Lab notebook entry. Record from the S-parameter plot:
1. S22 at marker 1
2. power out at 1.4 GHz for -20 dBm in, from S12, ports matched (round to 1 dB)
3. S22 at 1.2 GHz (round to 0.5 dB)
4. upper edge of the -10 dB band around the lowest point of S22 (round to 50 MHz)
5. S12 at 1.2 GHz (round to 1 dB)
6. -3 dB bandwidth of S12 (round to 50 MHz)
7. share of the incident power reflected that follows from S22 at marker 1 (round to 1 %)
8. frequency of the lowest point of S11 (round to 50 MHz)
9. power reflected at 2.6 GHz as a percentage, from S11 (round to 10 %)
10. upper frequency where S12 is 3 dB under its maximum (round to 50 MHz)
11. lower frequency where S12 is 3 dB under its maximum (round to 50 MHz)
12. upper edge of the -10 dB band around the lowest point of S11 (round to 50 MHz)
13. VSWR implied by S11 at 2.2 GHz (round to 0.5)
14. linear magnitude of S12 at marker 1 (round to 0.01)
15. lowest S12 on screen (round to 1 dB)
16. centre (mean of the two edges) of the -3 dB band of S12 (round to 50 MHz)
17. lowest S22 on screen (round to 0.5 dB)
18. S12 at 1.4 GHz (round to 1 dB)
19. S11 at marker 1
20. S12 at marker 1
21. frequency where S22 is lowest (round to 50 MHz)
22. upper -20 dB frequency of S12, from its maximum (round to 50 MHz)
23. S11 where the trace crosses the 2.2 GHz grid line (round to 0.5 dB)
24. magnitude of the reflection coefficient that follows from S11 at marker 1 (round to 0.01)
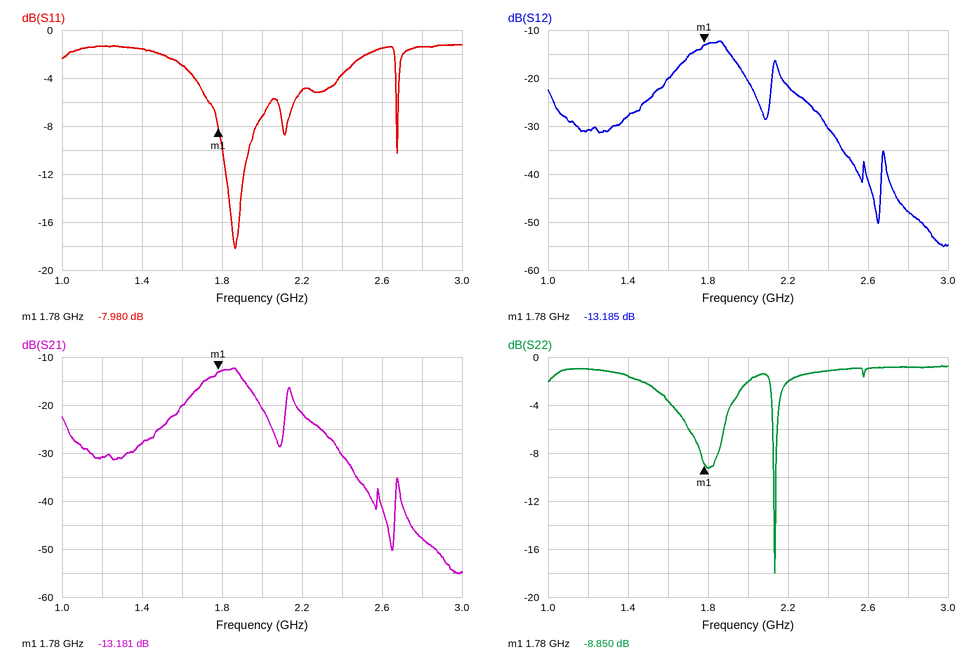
-8.850 dB
-48 dBm
-1.0 dB
2.15 GHz
-31 dB
200 MHz
13 %
1.85 GHz
70 %
1.90 GHz
1.70 GHz
1.95 GHz
3.5
0.22
-55 dB
1.80 GHz
-18.0 dB
-28 dB
-7.980 dB
-13.185 dB
2.15 GHz
2.45 GHz
-5.0 dB
0.40
